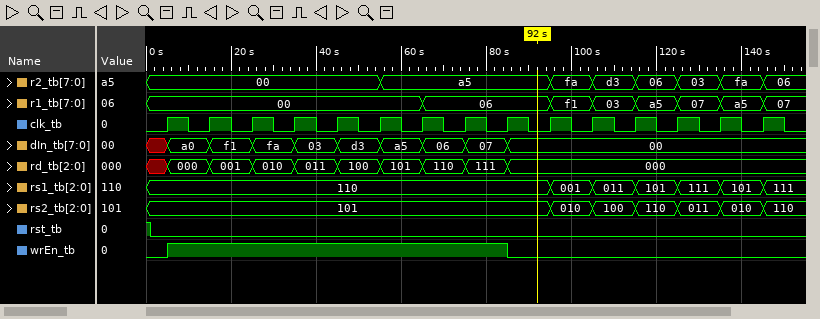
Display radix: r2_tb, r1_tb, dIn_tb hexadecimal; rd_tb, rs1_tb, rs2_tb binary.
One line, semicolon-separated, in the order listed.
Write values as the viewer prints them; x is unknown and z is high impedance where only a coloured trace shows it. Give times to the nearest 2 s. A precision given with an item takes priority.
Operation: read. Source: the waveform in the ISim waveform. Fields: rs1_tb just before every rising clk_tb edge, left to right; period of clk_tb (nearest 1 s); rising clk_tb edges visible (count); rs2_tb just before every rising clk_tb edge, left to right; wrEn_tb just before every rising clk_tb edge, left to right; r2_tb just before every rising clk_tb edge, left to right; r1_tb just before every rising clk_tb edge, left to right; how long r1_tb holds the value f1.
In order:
110, 110, 110, 110, 110, 110, 110, 110, 110, 110, 001, 011, 101, 111, 101; 10 s; 15; 101, 101, 101, 101, 101, 101, 101, 101, 101, 101, 010, 100, 110, 011, 010; 0 1 1 1 1 1 1 1 1 0 0 0 0 0 0; 00, 00, 00, 00, 00, 00, a5, a5, a5, a5, fa, d3, 06, 03, fa; 00, 00, 00, 00, 00, 00, 00, 06, 06, 06, f1, 03, a5, 07, a5; 10 s
